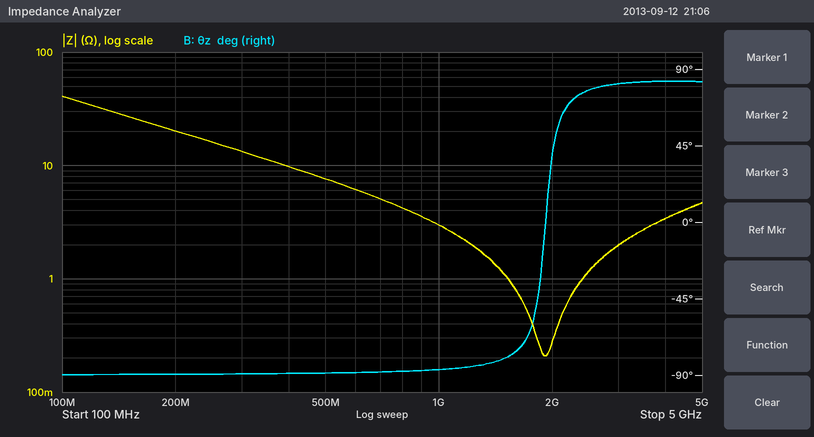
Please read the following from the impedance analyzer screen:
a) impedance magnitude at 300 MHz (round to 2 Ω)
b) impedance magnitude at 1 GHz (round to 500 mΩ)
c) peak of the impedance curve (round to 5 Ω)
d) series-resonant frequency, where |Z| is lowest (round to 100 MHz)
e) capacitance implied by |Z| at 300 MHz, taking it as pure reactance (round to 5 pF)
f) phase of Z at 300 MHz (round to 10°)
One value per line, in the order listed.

14 Ω
3.0 Ω
40 Ω
1.9 GHz
40 pF
-90°
